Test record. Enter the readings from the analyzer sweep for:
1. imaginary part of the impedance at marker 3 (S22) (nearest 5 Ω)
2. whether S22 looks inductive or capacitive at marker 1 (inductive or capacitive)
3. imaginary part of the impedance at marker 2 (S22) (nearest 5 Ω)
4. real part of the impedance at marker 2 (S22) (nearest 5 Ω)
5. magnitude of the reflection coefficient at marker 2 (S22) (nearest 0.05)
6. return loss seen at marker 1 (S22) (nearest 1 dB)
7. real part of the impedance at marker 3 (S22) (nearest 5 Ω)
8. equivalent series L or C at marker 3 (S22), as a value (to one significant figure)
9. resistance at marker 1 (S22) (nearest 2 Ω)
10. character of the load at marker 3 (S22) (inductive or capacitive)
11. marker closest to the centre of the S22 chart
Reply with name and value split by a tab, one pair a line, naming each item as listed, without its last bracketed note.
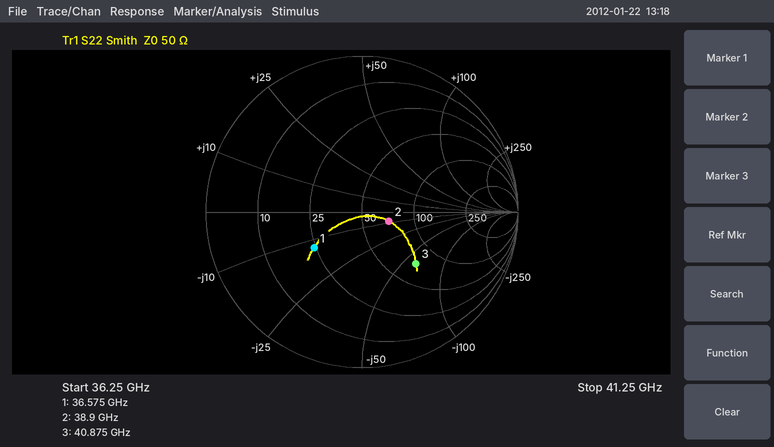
imaginary part of the impedance at marker 3 (S22)	-60 Ω
whether S22 looks inductive or capacitive at marker 1	capacitive
imaginary part of the impedance at marker 2 (S22)	-10 Ω
real part of the impedance at marker 2 (S22)	70 Ω
magnitude of the reflection coefficient at marker 2 (S22)	0.20
return loss seen at marker 1 (S22)	8 dB
real part of the impedance at marker 3 (S22)	70 Ω
equivalent series L or C at marker 3 (S22), as a value	60 fF
resistance at marker 1 (S22)	24 Ω
character of the load at marker 3 (S22)	capacitive
marker closest to the centre of the S22 chart	marker 2
